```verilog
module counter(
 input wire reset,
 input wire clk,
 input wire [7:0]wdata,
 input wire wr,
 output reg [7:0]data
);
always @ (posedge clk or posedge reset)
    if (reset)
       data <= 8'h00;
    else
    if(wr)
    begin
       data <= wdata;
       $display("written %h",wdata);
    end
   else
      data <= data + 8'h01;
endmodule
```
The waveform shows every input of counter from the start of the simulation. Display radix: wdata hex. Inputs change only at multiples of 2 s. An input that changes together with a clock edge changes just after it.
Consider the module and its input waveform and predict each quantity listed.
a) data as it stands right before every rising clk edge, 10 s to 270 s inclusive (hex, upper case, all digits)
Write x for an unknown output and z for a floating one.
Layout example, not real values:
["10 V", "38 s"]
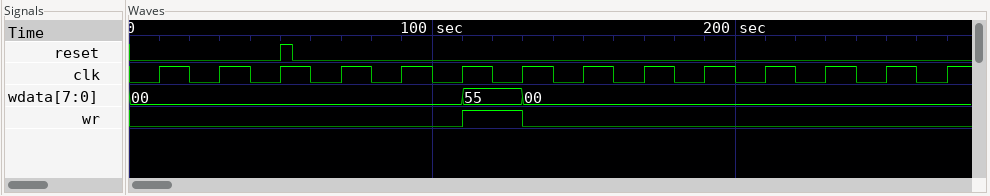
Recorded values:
["x, x, x, 00, 01, 02, 03, 55, 56, 57, 58, 59, 5A, 5B"]
